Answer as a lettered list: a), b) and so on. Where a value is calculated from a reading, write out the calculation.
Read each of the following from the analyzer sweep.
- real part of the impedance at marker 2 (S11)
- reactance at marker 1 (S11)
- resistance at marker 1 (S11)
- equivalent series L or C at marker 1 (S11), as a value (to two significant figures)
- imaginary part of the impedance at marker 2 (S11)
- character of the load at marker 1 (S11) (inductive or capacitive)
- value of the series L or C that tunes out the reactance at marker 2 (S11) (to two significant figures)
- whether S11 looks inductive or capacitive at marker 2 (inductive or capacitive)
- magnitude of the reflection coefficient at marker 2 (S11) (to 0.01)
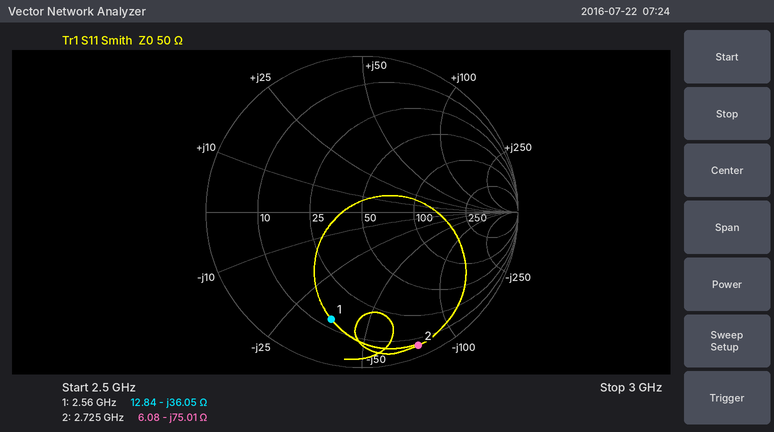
a) 6.08 Ω
b) -36.05 Ω
c) 12.84 Ω
d) C = 1/(2π × 2.56 GHz × 36.05 Ω) ≈ 1.7 pF
e) -75.01 Ω
f) capacitive
g) L = 75.01 Ω/(2π × 2.725 GHz) ≈ 4.4 nH
h) capacitive
i) 0.93
